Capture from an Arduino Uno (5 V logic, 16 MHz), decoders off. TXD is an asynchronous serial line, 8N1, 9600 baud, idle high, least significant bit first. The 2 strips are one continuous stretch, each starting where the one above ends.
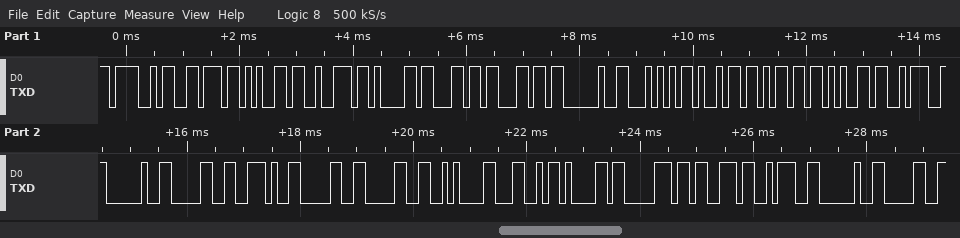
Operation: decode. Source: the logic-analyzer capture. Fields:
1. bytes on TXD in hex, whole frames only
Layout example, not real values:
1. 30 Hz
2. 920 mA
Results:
1. 0x4F 0x76 0x65 0x72 0x61 0x6C 0x6C 0x20 0x54 0x69 0x6D 0x65 0x3A 0x20 0x30 0x2E 0x30 0x30 0x0A 0x4C 0x61 0x70 0x73 0x3A 0x20 0x30
